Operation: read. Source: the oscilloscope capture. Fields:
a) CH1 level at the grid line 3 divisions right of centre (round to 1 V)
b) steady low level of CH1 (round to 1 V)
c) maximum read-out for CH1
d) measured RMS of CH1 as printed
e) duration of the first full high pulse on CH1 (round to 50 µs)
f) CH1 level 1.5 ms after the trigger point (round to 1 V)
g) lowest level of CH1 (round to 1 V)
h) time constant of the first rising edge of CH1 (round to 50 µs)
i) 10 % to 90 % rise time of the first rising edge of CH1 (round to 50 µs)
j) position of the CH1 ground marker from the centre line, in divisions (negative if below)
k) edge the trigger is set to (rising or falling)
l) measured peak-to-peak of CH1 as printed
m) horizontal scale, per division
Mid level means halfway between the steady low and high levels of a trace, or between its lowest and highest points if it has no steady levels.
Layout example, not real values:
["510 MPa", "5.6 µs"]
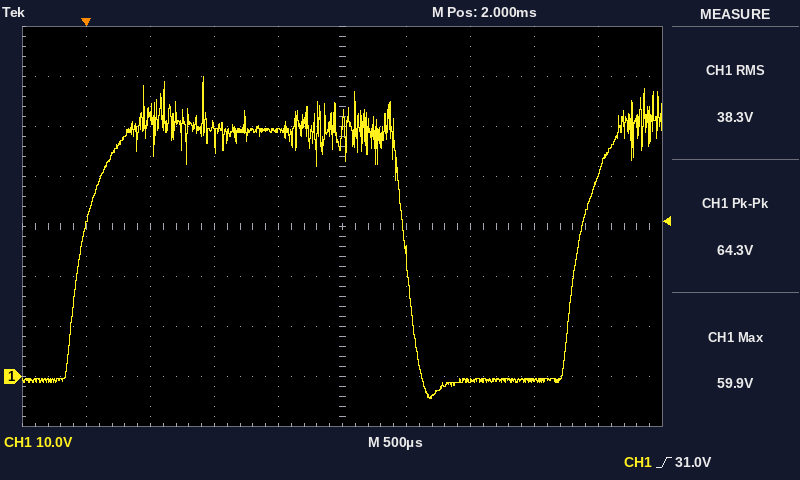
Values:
["-1 V", "-1 V", "59.9 V", "38.3 V", "2.55 ms", "49 V", "-4 V", "150 µs", "350 µs", "-3.0 div", "rising", "64.3 V", "500 µs"]
